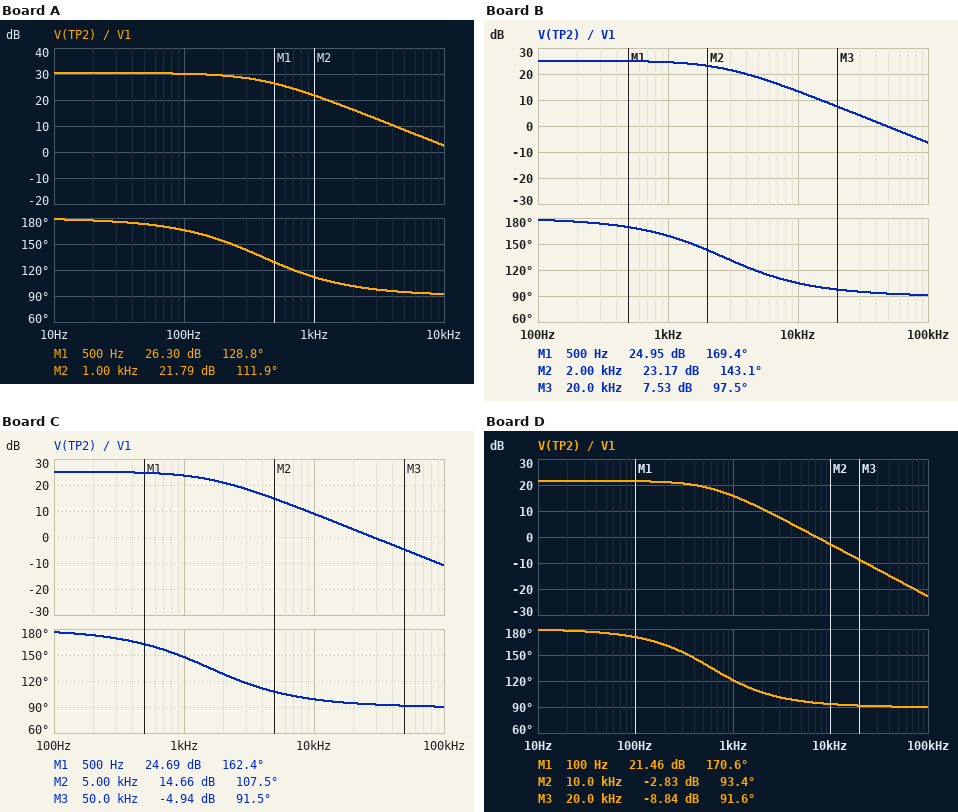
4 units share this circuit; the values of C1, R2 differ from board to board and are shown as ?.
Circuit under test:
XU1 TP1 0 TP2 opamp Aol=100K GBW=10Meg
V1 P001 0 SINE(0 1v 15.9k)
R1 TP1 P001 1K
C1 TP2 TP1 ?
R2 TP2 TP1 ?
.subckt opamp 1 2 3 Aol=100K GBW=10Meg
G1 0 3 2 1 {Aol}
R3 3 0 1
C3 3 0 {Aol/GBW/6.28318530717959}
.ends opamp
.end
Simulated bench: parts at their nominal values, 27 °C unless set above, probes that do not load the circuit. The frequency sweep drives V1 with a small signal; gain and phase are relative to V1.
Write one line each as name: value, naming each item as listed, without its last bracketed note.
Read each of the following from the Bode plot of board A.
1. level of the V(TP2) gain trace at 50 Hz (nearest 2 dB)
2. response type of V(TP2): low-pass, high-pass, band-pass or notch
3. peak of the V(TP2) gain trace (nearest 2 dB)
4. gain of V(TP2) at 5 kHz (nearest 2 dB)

level of the V(TP2) gain trace at 50 Hz: 30 dB
response type of V(TP2): low-pass, high-pass, band-pass or notch: low-pass
peak of the V(TP2) gain trace: 30 dB
gain of V(TP2) at 5 kHz: 8 dB
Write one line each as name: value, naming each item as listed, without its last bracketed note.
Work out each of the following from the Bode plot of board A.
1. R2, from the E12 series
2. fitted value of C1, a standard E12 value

R2, from the E12 series: 33 kΩ
fitted value of C1, a standard E12 value: 12 nF
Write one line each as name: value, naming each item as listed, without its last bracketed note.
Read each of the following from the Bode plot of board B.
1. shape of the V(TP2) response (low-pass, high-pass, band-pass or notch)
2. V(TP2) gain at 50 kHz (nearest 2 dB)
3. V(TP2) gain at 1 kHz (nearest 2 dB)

shape of the V(TP2) response: low-pass
V(TP2) gain at 50 kHz: 0 dB
V(TP2) gain at 1 kHz: 24 dB
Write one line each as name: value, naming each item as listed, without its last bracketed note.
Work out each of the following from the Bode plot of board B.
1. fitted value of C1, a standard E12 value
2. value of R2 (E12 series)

fitted value of C1, a standard E12 value: 3.3 nF
value of R2: 18 kΩ
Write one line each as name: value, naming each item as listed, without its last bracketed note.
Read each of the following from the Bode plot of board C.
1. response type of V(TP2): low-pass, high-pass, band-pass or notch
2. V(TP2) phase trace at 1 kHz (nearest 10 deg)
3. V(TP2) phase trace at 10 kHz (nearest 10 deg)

response type of V(TP2): low-pass, high-pass, band-pass or notch: low-pass
V(TP2) phase trace at 1 kHz: 150 deg
V(TP2) phase trace at 10 kHz: 100 deg
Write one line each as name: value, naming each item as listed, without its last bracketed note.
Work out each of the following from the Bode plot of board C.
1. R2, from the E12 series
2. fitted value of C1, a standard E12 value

R2, from the E12 series: 18 kΩ
fitted value of C1, a standard E12 value: 5.6 nF
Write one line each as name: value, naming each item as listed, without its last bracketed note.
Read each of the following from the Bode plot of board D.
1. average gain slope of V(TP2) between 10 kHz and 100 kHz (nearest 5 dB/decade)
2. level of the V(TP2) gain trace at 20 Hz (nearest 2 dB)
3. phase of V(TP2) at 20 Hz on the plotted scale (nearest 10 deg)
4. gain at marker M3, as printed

average gain slope of V(TP2) between 10 kHz and 100 kHz: -20 dB/decade
level of the V(TP2) gain trace at 20 Hz: 22 dB
phase of V(TP2) at 20 Hz on the plotted scale: 180 deg
gain at marker M3, as printed: -8.84 dB
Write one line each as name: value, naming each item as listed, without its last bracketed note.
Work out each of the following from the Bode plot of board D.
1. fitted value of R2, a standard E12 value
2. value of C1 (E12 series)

fitted value of R2, a standard E12 value: 12 kΩ
value of C1: 22 nF
